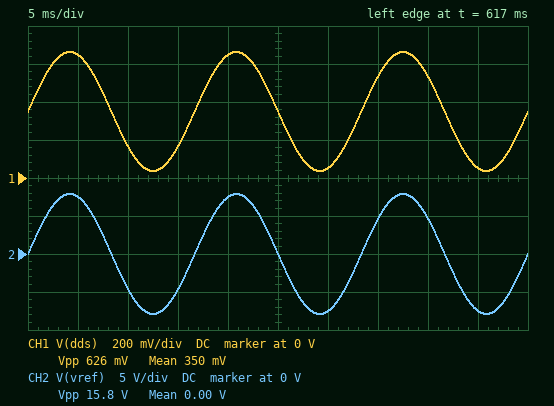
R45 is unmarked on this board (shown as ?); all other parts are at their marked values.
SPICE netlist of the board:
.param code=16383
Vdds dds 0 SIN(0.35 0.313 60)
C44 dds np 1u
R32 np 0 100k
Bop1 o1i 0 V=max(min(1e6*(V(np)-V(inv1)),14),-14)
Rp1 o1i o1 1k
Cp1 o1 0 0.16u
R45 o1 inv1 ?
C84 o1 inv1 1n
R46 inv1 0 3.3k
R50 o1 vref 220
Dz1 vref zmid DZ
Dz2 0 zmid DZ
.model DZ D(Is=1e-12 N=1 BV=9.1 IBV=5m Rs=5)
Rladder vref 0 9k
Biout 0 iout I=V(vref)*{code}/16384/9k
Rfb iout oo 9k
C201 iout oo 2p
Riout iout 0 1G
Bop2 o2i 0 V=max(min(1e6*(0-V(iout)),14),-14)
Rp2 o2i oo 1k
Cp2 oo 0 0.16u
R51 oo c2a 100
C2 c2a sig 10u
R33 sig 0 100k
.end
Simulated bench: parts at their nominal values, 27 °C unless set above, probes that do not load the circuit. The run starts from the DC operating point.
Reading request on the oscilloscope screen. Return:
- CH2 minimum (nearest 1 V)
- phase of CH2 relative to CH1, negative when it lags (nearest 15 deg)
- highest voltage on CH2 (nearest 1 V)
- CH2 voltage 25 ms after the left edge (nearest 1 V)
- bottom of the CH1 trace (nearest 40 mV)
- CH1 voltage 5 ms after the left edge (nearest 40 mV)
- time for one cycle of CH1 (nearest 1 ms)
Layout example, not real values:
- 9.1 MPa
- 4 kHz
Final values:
- -8 V
- 0 deg
- 8 V
- 0 V
- 40 mV
- 640 mV
- 17 ms
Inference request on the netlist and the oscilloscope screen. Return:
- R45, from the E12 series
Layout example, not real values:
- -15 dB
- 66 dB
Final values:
- 82 kΩ
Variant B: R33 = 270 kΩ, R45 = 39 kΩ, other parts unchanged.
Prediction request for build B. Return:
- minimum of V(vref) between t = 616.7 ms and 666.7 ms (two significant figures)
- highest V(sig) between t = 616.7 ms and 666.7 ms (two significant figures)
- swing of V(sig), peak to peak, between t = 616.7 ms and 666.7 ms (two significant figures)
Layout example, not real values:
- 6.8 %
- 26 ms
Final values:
- -3.9 V
- 3.9 V
- 7.8 V
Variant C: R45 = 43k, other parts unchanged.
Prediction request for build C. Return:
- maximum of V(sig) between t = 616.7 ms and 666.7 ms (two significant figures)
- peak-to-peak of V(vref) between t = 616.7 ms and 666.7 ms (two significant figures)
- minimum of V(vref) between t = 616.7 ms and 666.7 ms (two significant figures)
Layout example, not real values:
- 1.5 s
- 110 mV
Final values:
- 4.3 V
- 8.6 V
- -4.3 V
